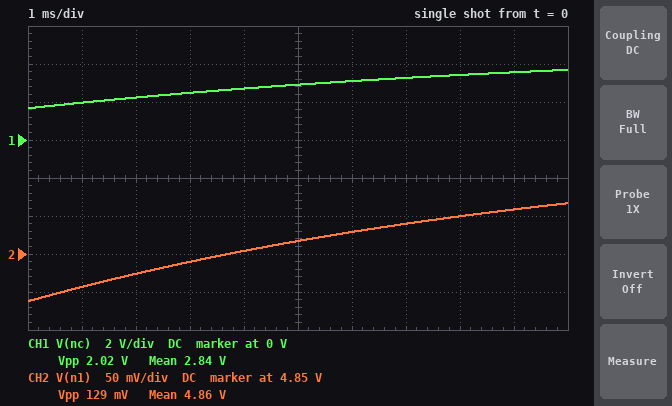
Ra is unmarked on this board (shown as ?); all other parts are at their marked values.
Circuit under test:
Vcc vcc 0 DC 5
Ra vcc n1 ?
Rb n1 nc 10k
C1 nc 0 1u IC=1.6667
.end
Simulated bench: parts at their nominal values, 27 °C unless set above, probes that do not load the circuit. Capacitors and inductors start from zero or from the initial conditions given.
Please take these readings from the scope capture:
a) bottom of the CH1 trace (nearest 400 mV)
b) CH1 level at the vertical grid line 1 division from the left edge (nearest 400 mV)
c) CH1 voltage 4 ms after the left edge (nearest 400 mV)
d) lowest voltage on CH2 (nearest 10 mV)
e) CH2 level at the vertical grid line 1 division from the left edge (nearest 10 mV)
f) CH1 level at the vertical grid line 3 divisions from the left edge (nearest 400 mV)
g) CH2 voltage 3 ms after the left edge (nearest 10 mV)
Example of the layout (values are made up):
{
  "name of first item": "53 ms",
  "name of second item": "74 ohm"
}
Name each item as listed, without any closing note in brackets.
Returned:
{
  "bottom of the CH1 trace": "1.6 V",
  "CH1 level at the vertical grid line 1 division from the left edge": "2.0 V",
  "CH1 voltage 4 ms after the left edge": "2.8 V",
  "lowest voltage on CH2": "4.79 V",
  "CH2 level at the vertical grid line 1 division from the left edge": "4.81 V",
  "CH1 level at the vertical grid line 3 divisions from the left edge": "2.4 V",
  "CH2 voltage 3 ms after the left edge": "4.84 V"
}
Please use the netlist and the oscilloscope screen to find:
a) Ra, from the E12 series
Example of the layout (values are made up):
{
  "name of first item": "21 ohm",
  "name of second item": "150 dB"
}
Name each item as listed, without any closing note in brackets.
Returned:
{
  "Ra, from the E12 series": "680 Ω"
}
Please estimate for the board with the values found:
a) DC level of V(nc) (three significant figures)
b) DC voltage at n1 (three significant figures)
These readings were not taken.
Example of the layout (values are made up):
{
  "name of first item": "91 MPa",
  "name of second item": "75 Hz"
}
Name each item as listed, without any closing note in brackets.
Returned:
{
  "DC level of V(nc)": "5.00 V",
  "DC voltage at n1": "5.00 V"
}
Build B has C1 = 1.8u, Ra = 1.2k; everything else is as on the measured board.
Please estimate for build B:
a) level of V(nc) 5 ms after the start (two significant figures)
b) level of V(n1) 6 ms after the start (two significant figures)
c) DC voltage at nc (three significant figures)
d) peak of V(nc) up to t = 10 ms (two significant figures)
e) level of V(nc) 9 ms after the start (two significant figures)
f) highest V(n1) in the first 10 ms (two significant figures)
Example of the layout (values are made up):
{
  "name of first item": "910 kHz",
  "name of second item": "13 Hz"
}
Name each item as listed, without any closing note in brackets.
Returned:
{
  "level of V(nc) 5 ms after the start": "2.4 V",
  "level of V(n1) 6 ms after the start": "4.7 V",
  "DC voltage at nc": "5.00 V",
  "peak of V(nc) up to t = 10 ms": "3.0 V",
  "level of V(nc) 9 ms after the start": "2.9 V",
  "highest V(n1) in the first 10 ms": "4.8 V"
}
